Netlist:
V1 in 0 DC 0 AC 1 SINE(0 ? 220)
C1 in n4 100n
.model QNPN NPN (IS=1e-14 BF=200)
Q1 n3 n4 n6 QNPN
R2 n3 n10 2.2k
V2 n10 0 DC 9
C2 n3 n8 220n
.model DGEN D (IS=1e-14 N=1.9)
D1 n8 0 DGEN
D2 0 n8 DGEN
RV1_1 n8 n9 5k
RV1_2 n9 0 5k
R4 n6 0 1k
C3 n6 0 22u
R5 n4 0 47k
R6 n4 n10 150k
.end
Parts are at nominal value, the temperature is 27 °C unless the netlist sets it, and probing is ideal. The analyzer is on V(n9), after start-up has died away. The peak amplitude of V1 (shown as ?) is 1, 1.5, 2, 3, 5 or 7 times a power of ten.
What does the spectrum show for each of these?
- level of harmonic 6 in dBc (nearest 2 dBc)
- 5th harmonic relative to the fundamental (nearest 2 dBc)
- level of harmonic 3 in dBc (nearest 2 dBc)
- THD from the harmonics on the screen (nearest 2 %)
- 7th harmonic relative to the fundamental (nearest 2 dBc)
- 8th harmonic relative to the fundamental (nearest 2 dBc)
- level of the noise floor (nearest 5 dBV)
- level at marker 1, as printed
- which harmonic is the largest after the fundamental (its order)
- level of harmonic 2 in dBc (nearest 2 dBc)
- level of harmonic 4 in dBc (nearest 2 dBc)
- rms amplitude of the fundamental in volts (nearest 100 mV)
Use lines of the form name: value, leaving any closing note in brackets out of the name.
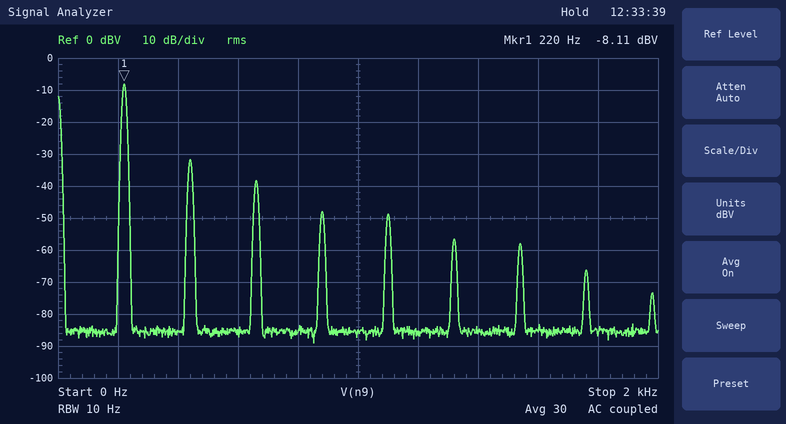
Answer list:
level of harmonic 6 in dBc: -48 dBc
5th harmonic relative to the fundamental: -40 dBc
level of harmonic 3 in dBc: -30 dBc
THD from the harmonics on the screen: 8 %
7th harmonic relative to the fundamental: -50 dBc
8th harmonic relative to the fundamental: -58 dBc
level of the noise floor: -85 dBV
level at marker 1, as printed: -8.11 dBV
which harmonic is the largest after the fundamental: 2
level of harmonic 2 in dBc: -24 dBc
level of harmonic 4 in dBc: -40 dBc
rms amplitude of the fundamental in volts: 400 mV
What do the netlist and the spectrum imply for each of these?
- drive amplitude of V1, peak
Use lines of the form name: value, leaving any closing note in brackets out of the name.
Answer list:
drive amplitude of V1, peak: 50 mV
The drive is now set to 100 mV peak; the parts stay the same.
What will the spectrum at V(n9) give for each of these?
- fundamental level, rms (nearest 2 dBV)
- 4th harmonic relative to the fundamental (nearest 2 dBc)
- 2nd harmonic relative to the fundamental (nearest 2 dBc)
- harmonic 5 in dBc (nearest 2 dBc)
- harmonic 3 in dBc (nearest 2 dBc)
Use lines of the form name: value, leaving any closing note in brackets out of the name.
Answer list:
fundamental level, rms: -6 dBV
4th harmonic relative to the fundamental: -22 dBc
2nd harmonic relative to the fundamental: -14 dBc
harmonic 5 in dBc: -30 dBc
harmonic 3 in dBc: -16 dBc
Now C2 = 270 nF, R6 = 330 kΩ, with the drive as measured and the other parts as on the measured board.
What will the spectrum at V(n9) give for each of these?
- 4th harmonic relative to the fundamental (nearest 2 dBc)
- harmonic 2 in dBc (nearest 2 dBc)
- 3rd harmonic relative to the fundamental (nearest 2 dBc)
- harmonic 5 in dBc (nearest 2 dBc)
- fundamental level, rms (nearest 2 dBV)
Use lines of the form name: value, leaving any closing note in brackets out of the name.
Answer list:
4th harmonic relative to the fundamental: -34 dBc
harmonic 2 in dBc: -12 dBc
3rd harmonic relative to the fundamental: -24 dBc
harmonic 5 in dBc: -42 dBc
fundamental level, rms: -12 dBV
